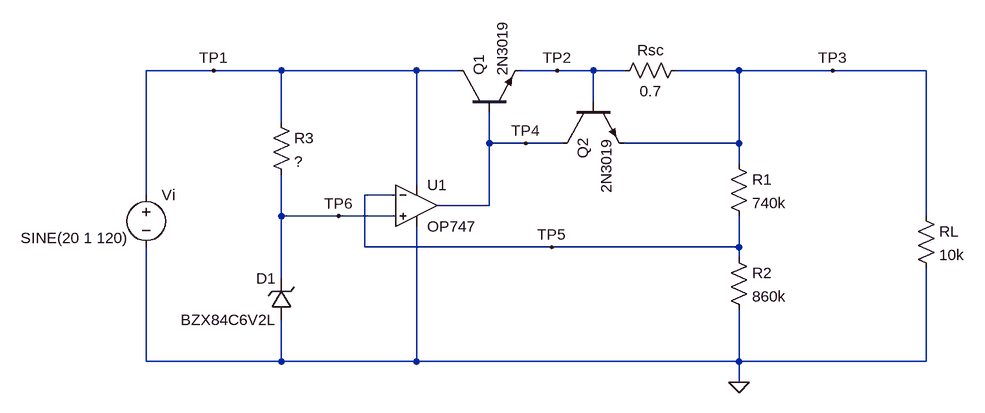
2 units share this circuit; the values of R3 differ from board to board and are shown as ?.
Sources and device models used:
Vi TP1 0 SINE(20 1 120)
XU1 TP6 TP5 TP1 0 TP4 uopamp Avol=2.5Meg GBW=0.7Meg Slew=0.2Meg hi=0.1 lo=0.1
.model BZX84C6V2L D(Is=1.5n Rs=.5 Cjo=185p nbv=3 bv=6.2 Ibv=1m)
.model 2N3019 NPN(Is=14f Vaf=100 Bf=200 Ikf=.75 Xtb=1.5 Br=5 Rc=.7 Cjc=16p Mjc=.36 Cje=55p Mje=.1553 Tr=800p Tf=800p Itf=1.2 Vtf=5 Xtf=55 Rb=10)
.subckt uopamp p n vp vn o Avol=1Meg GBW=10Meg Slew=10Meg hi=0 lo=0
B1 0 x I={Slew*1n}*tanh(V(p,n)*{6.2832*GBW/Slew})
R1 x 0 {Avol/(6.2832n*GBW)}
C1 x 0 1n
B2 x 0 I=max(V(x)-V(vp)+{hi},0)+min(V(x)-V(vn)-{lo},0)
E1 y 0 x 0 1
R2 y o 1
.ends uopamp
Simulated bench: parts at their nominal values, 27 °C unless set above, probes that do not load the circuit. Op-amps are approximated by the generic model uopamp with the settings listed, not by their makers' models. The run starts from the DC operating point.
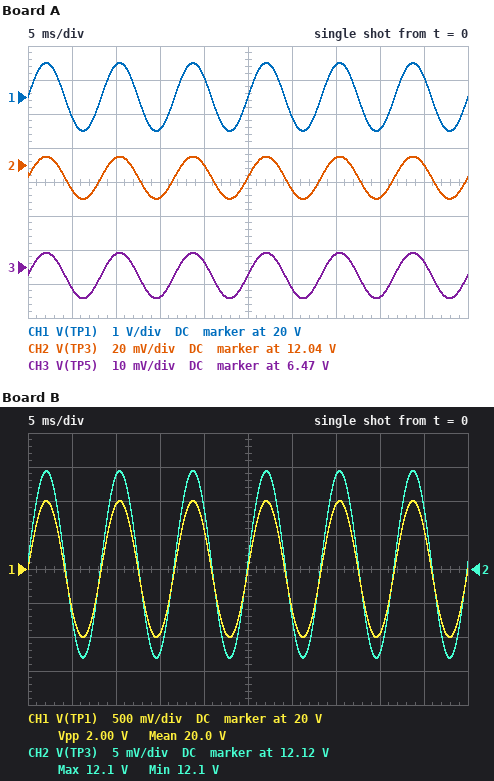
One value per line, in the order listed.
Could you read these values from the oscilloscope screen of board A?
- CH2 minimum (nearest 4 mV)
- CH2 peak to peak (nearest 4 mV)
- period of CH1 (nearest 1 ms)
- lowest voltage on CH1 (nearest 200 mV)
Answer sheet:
12.020 V
24 mV
8 ms
19.0 V
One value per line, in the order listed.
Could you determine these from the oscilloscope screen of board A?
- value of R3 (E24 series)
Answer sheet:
510 Ω
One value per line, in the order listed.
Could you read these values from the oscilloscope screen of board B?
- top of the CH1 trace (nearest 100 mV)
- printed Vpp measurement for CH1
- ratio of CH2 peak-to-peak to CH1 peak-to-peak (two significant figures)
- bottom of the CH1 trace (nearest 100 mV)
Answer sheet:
21.0 V
2.00 V
0.014
19.0 V
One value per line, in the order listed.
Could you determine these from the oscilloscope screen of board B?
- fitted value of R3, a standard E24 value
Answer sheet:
300 Ω
